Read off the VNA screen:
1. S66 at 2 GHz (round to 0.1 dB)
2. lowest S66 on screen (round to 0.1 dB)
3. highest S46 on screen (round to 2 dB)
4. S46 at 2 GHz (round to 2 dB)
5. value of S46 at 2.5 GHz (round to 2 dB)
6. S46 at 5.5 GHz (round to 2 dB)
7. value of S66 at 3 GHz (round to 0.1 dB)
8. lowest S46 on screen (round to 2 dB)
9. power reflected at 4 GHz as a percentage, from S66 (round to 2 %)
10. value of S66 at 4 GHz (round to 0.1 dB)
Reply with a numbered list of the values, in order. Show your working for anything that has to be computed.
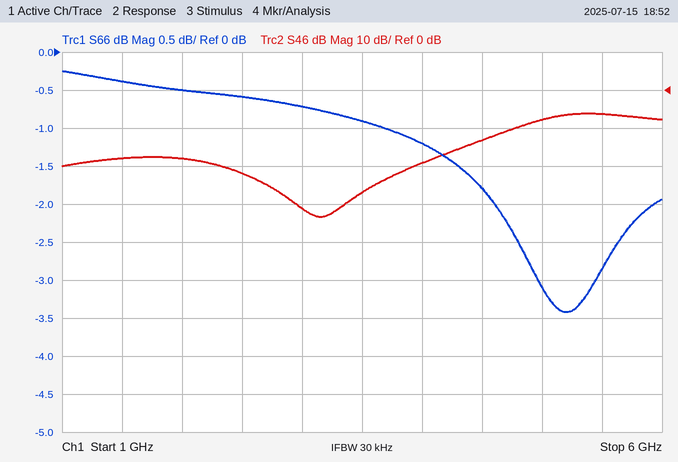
1. -0.5 dB
2. -3.4 dB
3. -6 dB
4. -18 dB
5. -22 dB
6. -6 dB
7. -0.7 dB
8. -34 dB
9. 10^(-1.2/10) ≈ 76 %
10. -1.2 dB
